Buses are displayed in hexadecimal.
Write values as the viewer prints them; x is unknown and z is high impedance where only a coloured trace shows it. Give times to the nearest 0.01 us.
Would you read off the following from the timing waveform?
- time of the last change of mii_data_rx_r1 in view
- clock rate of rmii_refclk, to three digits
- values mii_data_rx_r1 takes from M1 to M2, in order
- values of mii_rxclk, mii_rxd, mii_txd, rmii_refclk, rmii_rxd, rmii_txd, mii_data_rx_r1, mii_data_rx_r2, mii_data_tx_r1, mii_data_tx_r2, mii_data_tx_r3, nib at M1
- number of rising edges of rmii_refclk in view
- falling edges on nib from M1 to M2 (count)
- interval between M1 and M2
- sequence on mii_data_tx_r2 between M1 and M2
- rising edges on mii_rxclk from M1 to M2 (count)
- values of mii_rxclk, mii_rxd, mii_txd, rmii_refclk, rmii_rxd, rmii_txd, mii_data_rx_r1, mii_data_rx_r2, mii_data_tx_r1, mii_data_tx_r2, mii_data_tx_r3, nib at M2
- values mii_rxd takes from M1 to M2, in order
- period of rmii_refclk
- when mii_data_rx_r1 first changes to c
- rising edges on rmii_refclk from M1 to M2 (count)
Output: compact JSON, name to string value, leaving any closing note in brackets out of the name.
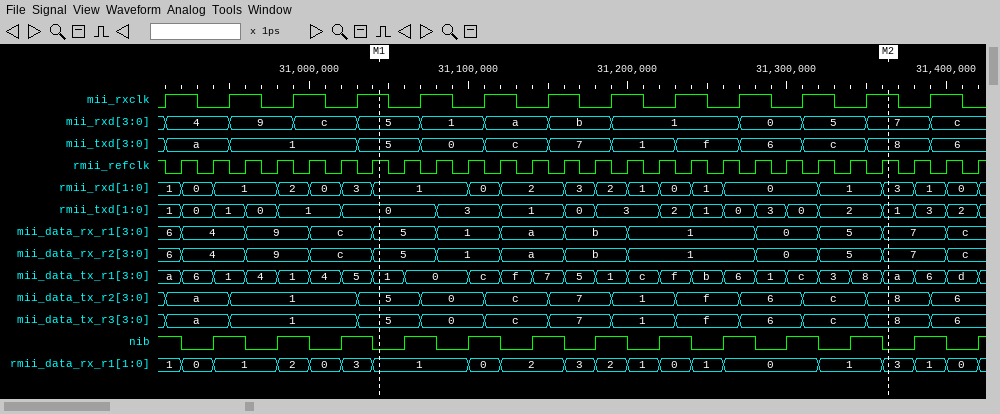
{"time of the last change of mii_data_rx_r1 in view": "31.4 us", "clock rate of rmii_refclk, to three digits": "50.0 MHz", "values mii_data_rx_r1 takes from M1 to M2, in order": "5, 1, a, b, 1, 0, 5, 7", "values of mii_rxclk, mii_rxd, mii_txd, rmii_refclk, rmii_rxd, rmii_txd, mii_data_rx_r1, mii_data_rx_r2, mii_data_tx_r1, mii_data_tx_r2, mii_data_tx_r3, nib at M1": "mii_rxclk=1, mii_rxd=5, mii_txd=5, rmii_refclk=1, rmii_rxd=1, rmii_txd=0, mii_data_rx_r1=5, mii_data_rx_r2=5, mii_data_tx_r1=1, mii_data_tx_r2=5, mii_data_tx_r3=5, nib=0", "number of rising edges of rmii_refclk in view": "26", "falling edges on nib from M1 to M2": "8", "interval between M1 and M2": "0.32 us", "sequence on mii_data_tx_r2 between M1 and M2": "5, 0, c, 7, 1, f, 6, c, 8", "rising edges on mii_rxclk from M1 to M2": "8", "values of mii_rxclk, mii_rxd, mii_txd, rmii_refclk, rmii_rxd, rmii_txd, mii_data_rx_r1, mii_data_rx_r2, mii_data_tx_r1, mii_data_tx_r2, mii_data_tx_r3, nib at M2": "mii_rxclk=1, mii_rxd=7, mii_txd=8, rmii_refclk=1, rmii_rxd=3, rmii_txd=1, mii_data_rx_r1=7, mii_data_rx_r2=7, mii_data_tx_r1=a, mii_data_tx_r2=8, mii_data_tx_r3=8, nib=0", "values mii_rxd takes from M1 to M2, in order": "5, 1, a, b, 1, 0, 5, 7", "period of rmii_refclk": "0.02 us", "when mii_data_rx_r1 first changes to c": "31 us", "rising edges on rmii_refclk from M1 to M2": "16"}
